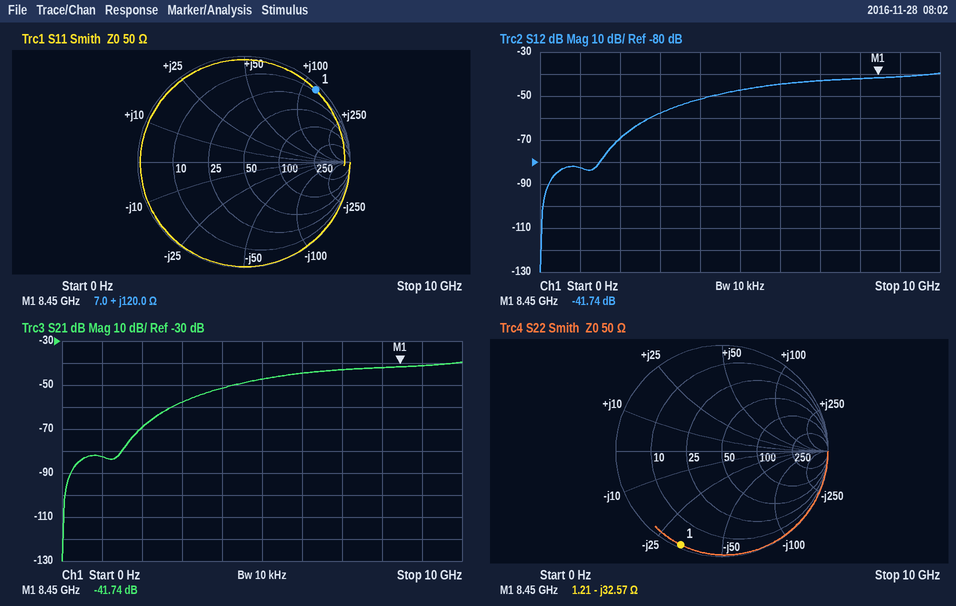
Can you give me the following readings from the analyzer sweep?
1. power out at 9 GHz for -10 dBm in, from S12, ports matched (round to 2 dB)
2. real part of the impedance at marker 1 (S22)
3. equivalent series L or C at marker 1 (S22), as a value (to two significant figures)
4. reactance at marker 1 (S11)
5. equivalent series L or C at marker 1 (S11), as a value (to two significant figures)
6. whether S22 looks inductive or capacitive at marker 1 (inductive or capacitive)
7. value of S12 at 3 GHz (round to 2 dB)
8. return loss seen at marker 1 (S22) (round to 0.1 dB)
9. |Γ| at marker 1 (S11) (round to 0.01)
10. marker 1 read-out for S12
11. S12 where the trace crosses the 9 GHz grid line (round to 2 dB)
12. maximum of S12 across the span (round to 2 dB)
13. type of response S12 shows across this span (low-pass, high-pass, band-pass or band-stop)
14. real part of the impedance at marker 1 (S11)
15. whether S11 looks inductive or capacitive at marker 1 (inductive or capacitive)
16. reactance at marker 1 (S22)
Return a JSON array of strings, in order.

["-52 dBm", "1.21 Ω", "580 fF", "+120.0 Ω", "2.3 nH", "capacitive", "-58 dB", "0.3 dB", "0.96", "-41.74 dB", "-42 dB", "-40 dB", "high-pass", "7.0 Ω", "inductive", "-32.57 Ω"]
